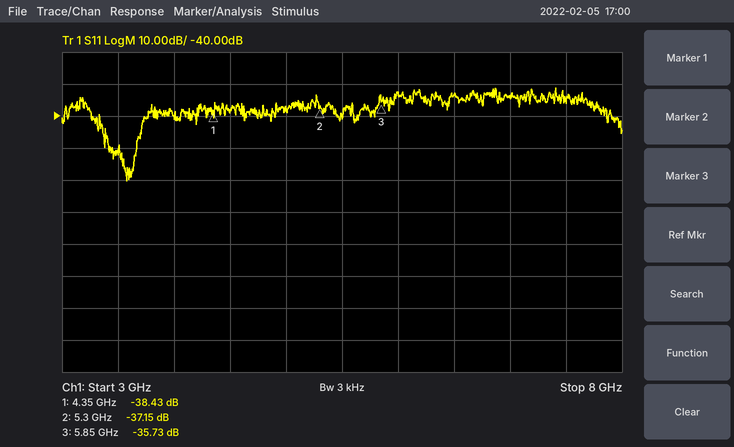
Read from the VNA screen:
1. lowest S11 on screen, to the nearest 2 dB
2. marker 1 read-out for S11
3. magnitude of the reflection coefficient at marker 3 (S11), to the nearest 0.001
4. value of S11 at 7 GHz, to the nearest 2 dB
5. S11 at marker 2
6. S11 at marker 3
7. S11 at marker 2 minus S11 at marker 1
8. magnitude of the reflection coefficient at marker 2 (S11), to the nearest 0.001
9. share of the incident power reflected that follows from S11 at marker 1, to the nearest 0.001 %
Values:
-60 dB
-38.43 dB
0.016
-34 dB
-37.15 dB
-35.73 dB
1.28 dB
0.014
0.014 %
